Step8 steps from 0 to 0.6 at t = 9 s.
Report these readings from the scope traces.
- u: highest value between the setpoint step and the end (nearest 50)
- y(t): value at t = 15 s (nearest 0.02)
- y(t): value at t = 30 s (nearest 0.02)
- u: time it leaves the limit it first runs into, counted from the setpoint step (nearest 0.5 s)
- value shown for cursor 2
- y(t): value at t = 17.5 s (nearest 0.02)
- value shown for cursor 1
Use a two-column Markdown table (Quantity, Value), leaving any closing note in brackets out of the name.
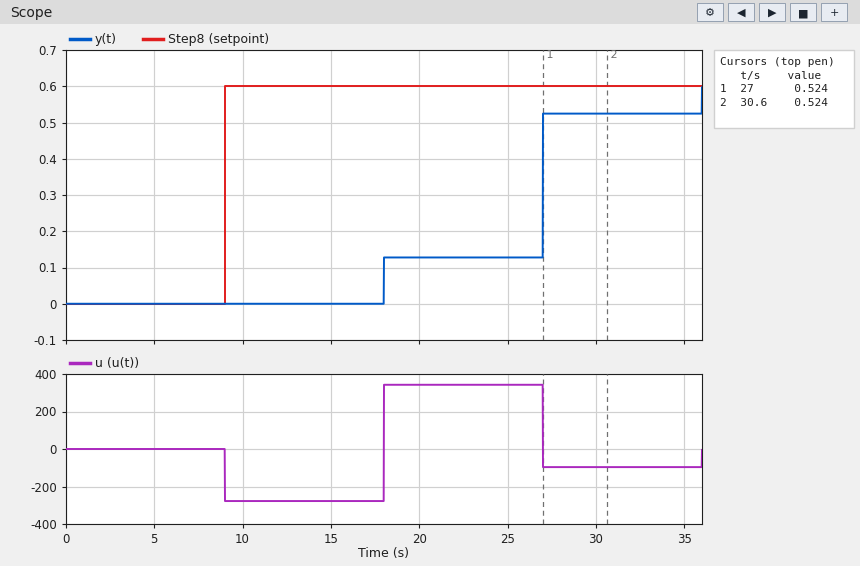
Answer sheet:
| Quantity | Value |
|---|---|
| u: highest value between the setpoint step and the end | 350 |
| y(t): value at t = 15 s | 0.00 |
| y(t): value at t = 30 s | 0.52 |
| u: time it leaves the limit it first runs into, counted from the setpoint step | 9.0 s |
| value shown for cursor 2 | 0.524 |
| y(t): value at t = 17.5 s | 0.00 |
| value shown for cursor 1 | 0.524 |
